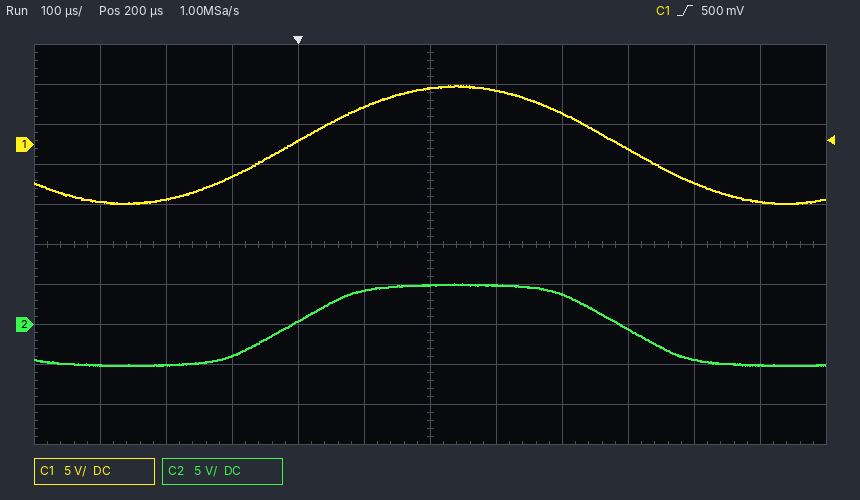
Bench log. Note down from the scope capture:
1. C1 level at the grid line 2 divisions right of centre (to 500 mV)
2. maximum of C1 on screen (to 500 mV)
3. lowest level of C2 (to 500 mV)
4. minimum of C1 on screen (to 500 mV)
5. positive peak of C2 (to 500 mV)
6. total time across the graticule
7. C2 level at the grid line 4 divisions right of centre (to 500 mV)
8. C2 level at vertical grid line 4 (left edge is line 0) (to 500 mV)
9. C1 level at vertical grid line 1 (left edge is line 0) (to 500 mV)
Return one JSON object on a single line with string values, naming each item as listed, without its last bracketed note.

{"C1 level at the grid line 2 divisions right of centre": "4.0 V", "maximum of C1 on screen": "7.5 V", "lowest level of C2": "-5.0 V", "minimum of C1 on screen": "-7.5 V", "positive peak of C2": "5.0 V", "total time across the graticule": "1.2 ms", "C2 level at the grid line 4 divisions right of centre": "-4.5 V", "C2 level at vertical grid line 4 (left edge is line 0)": "500 mV", "C1 level at vertical grid line 1 (left edge is line 0)": "-7.0 V"}
